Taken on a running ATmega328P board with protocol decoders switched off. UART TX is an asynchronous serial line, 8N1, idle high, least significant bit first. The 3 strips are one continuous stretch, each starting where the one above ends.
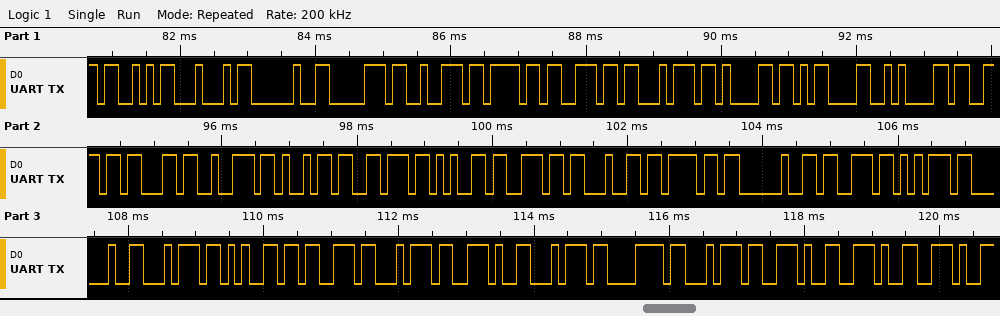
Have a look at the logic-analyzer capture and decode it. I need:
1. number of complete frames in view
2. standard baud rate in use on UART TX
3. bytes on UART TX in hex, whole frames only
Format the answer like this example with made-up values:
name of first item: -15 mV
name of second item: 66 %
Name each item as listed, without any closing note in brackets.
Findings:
number of complete frames in view: 35
standard baud rate in use on UART TX: 9600 baud
bytes on UART TX in hex, whole frames only: 0x53 0x44 0x20 0x70 0x72 0x6F 0x6E 0x74 0x61 0x0D 0x0A 0x73 0x63 0x72 0x69 0x76 0x65 0x6E 0x64 0x6F 0x20 0x73 0x75 0x20 0x74 0x65 0x73 0x74 0x2E 0x74 0x78 0x74 0x2E 0x2E 0x2E
